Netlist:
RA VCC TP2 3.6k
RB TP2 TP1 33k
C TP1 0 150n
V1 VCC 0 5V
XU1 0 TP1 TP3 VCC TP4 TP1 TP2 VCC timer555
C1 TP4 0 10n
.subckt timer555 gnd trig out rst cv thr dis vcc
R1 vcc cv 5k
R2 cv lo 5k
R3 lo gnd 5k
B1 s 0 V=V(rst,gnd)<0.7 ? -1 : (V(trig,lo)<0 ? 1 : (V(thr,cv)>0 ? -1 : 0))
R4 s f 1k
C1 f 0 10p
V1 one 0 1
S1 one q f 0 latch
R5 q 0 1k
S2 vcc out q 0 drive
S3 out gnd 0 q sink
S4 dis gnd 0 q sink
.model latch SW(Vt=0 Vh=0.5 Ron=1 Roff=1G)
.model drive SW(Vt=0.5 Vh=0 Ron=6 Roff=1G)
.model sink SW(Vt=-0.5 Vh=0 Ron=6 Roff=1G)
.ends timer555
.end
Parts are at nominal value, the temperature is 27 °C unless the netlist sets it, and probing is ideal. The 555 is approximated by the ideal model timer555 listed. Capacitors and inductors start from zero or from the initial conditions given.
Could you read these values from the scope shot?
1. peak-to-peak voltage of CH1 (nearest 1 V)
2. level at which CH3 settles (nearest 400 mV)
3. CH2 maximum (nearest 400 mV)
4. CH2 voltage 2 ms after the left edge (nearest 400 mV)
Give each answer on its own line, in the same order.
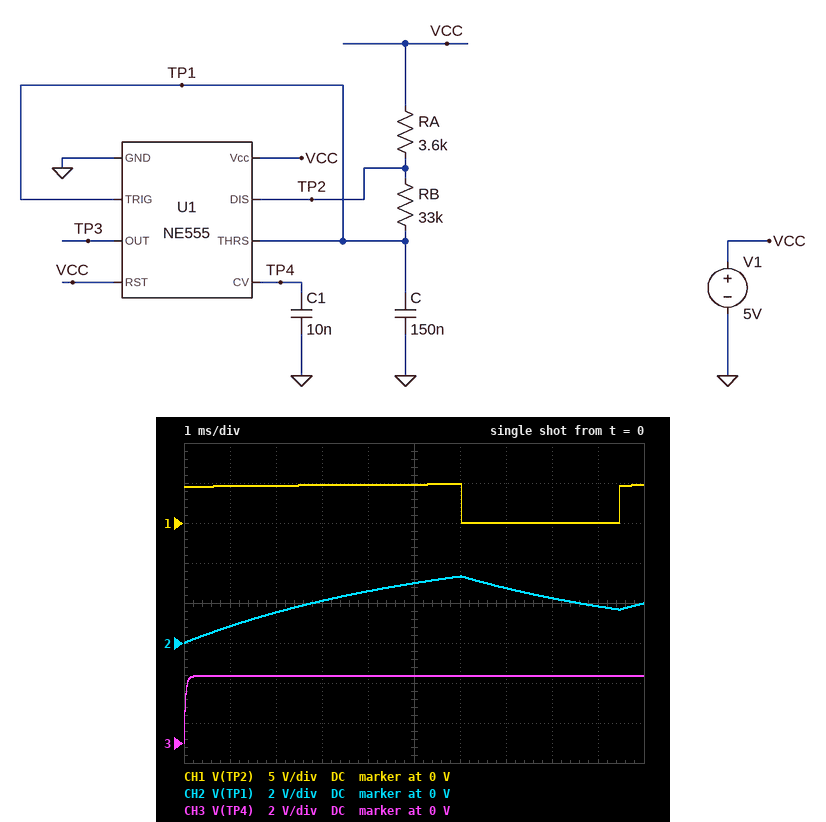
5 V
3.2 V
3.2 V
1.6 V
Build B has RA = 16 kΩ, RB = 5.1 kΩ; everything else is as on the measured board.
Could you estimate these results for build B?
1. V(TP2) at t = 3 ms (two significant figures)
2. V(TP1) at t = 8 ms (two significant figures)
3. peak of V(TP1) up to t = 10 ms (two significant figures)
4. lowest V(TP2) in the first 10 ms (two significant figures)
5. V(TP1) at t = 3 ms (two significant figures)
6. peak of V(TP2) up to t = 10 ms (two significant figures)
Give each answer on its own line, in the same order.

3.5 V
2.8 V
3.3 V
3.8 mV
3.1 V
3.7 V
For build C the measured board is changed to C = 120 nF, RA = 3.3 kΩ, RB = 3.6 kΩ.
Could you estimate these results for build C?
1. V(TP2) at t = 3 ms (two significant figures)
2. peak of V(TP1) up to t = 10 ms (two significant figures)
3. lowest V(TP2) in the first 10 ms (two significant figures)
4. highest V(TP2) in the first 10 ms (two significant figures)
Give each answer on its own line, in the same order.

3.5 V
3.3 V
12 mV
4.2 V
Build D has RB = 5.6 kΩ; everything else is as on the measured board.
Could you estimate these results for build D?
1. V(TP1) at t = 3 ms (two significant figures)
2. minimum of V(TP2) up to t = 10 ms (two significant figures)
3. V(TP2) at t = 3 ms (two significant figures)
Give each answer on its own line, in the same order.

3.3 V
10 mV
4.3 V
